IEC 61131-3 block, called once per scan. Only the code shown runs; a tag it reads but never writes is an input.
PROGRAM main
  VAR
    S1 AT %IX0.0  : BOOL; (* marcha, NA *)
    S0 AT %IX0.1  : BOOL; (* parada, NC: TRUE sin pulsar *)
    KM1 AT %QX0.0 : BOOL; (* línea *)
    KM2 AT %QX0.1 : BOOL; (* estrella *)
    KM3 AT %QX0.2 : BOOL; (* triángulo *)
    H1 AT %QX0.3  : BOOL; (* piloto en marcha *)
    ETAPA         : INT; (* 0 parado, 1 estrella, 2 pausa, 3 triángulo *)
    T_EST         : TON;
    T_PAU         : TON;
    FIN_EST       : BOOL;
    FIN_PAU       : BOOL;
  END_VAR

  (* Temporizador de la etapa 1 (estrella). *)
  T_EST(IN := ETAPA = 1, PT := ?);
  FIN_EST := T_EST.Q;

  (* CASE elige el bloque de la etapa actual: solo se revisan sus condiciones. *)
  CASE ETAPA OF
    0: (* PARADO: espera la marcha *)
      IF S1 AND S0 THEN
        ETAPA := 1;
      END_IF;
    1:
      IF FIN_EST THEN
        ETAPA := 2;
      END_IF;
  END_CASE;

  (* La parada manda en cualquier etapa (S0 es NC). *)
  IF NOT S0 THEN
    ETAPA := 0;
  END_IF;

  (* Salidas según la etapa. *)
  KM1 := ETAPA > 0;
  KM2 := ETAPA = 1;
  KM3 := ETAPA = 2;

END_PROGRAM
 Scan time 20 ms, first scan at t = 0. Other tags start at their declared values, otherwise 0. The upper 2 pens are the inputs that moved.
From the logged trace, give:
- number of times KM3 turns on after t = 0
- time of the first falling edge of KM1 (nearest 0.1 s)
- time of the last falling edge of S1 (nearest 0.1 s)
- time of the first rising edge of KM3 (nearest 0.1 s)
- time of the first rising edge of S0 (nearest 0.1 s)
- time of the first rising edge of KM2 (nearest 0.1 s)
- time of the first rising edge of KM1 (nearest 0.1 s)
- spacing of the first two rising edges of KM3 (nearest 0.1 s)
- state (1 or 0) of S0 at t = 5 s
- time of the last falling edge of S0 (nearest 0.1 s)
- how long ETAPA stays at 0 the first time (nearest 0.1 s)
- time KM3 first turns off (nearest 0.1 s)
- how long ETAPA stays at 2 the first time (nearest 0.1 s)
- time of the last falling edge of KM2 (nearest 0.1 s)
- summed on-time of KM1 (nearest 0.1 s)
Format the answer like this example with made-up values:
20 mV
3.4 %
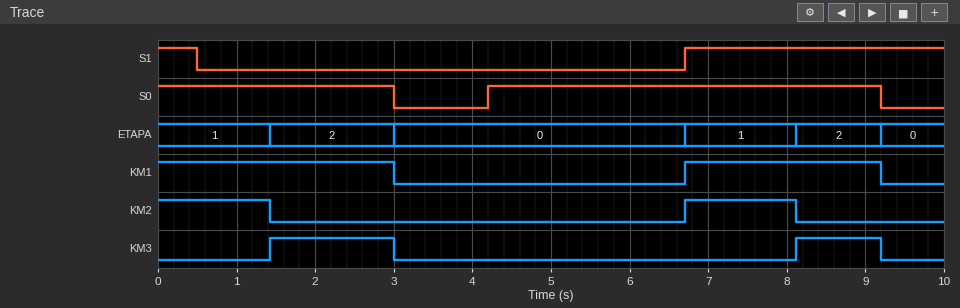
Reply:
2
3.0 s
0.5 s
1.4 s
4.2 s
6.7 s
6.7 s
6.7 s
1
9.2 s
3.7 s
3.0 s
1.6 s
8.1 s
5.5 s
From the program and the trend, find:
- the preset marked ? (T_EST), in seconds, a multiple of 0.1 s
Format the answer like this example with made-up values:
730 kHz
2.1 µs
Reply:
1.4 s
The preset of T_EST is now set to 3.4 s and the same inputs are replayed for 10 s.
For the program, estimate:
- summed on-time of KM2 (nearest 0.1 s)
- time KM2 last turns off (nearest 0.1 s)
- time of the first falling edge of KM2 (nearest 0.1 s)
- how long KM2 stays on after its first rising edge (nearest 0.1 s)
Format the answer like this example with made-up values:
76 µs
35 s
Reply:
5.5 s
9.2 s
3.0 s
2.5 s
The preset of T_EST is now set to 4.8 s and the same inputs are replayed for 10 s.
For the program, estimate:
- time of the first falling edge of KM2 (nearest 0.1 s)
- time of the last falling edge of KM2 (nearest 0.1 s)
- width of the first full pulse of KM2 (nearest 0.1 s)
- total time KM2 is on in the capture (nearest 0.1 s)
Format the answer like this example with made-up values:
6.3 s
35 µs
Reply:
3.0 s
9.2 s
2.5 s
5.5 s
